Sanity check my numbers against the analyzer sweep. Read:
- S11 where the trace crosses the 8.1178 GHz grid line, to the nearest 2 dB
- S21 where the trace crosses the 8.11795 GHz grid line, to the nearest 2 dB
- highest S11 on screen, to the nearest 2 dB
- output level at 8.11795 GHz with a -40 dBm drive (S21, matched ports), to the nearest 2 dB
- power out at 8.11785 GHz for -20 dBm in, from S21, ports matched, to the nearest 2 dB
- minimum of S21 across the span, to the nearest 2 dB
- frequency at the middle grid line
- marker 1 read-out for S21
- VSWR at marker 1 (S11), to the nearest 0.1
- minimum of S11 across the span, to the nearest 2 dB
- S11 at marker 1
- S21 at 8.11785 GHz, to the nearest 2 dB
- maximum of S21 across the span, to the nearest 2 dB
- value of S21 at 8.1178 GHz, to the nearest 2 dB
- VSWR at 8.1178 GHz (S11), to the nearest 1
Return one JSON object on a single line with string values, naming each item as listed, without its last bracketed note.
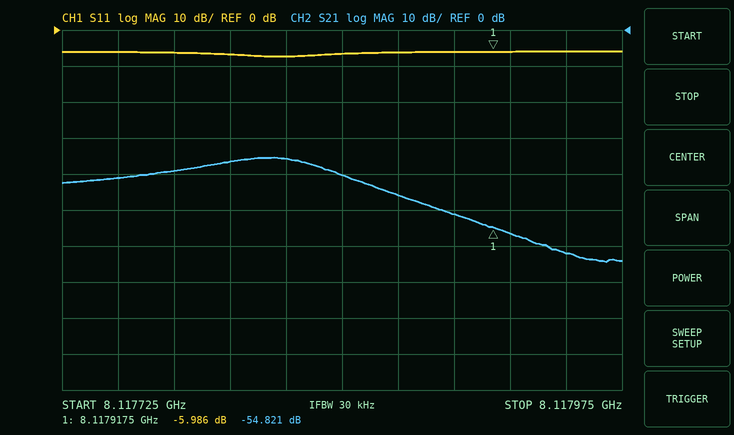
{"S11 where the trace crosses the 8.1178 GHz grid line, to the nearest 2 dB": "-6 dB", "S21 where the trace crosses the 8.11795 GHz grid line, to the nearest 2 dB": "-62 dB", "highest S11 on screen, to the nearest 2 dB": "-6 dB", "output level at 8.11795 GHz with a -40 dBm drive (S21, matched ports), to the nearest 2 dB": "-102 dBm", "power out at 8.11785 GHz for -20 dBm in, from S21, ports matched, to the nearest 2 dB": "-60 dBm", "minimum of S21 across the span, to the nearest 2 dB": "-64 dB", "frequency at the middle grid line": "8.11785 GHz", "marker 1 read-out for S21": "-54.821 dB", "VSWR at marker 1 (S11), to the nearest 0.1": "3.0", "minimum of S11 across the span, to the nearest 2 dB": "-8 dB", "S11 at marker 1": "-5.986 dB", "S21 at 8.11785 GHz, to the nearest 2 dB": "-40 dB", "maximum of S21 across the span, to the nearest 2 dB": "-36 dB", "value of S21 at 8.1178 GHz, to the nearest 2 dB": "-36 dB", "VSWR at 8.1178 GHz (S11), to the nearest 1": "3"}
